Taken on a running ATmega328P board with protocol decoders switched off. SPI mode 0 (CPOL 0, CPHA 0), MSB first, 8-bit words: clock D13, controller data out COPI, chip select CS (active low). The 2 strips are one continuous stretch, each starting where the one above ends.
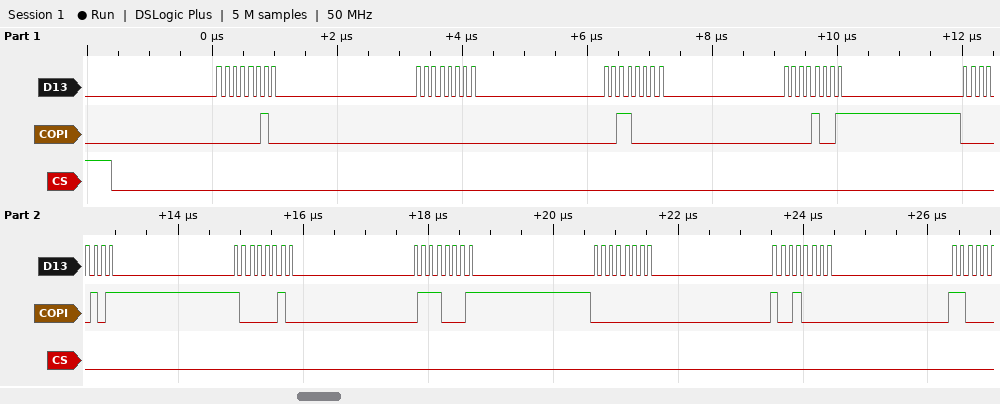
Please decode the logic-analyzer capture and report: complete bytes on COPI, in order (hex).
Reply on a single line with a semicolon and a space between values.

02 00 30 09 05 82 71 00 90
